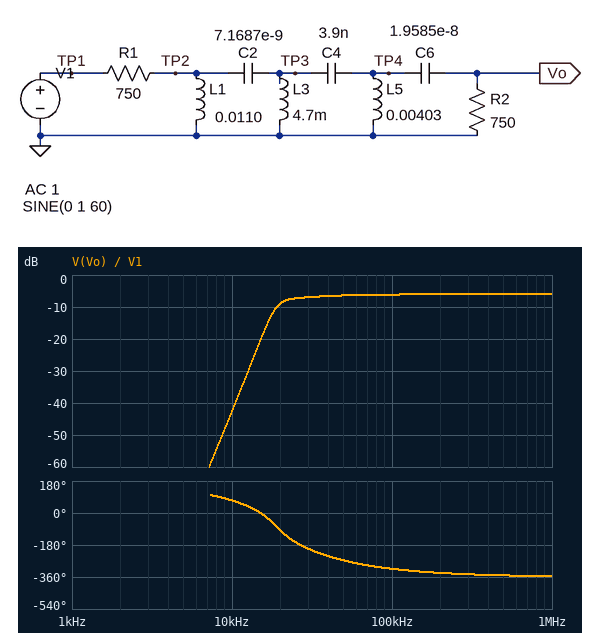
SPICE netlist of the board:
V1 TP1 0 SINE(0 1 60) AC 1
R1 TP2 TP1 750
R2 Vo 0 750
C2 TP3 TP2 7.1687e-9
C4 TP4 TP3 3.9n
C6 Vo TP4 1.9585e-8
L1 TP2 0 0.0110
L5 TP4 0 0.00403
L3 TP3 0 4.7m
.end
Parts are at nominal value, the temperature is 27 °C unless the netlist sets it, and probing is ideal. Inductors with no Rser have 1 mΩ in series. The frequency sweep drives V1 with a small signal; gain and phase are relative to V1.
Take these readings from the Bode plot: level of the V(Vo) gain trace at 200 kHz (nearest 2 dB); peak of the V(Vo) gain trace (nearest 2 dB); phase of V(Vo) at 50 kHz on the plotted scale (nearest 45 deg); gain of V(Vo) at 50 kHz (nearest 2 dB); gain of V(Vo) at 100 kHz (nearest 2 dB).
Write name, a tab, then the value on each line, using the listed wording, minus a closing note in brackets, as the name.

level of the V(Vo) gain trace at 200 kHz	-6 dB
peak of the V(Vo) gain trace	-6 dB
phase of V(Vo) at 50 kHz on the plotted scale	-270 deg
gain of V(Vo) at 50 kHz	-6 dB
gain of V(Vo) at 100 kHz	-6 dB
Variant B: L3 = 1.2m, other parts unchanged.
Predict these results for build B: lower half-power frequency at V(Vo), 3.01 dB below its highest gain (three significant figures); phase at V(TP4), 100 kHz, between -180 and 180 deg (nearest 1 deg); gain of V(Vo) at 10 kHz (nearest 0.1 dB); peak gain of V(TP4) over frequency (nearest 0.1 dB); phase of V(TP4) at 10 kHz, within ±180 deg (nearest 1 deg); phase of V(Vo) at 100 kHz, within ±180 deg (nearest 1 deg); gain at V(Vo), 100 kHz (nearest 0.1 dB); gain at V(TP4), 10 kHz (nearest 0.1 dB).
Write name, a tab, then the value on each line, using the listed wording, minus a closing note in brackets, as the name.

lower half-power frequency at V(Vo), 3.01 dB below its highest gain	41.8 kHz
phase at V(TP4), 100 kHz, between -180 and 180 deg	62 deg
gain of V(Vo) at 10 kHz	-56.2 dB
peak gain of V(TP4) over frequency	-6.0 dB
phase of V(TP4) at 10 kHz, within ±180 deg	25 deg
phase of V(Vo) at 100 kHz, within ±180 deg	68 deg
gain at V(Vo), 100 kHz	-6.3 dB
gain at V(TP4), 10 kHz	-52.8 dB
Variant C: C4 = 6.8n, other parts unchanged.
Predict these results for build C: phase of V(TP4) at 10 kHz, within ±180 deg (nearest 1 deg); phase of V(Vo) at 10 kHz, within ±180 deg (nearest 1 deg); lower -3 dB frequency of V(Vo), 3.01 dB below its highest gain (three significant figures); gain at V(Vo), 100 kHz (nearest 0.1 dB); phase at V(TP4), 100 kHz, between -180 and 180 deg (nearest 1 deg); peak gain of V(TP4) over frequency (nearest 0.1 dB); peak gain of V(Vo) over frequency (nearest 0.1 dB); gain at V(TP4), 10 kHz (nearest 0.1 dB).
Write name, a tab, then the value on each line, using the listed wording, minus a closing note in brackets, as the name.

phase of V(TP4) at 10 kHz, within ±180 deg	22 deg
phase of V(Vo) at 10 kHz, within ±180 deg	69 deg
lower -3 dB frequency of V(Vo), 3.01 dB below its highest gain	15.7 kHz
gain at V(Vo), 100 kHz	-6.0 dB
phase at V(TP4), 100 kHz, between -180 and 180 deg	33 deg
peak gain of V(TP4) over frequency	-4.8 dB
peak gain of V(Vo) over frequency	-6.0 dB
gain at V(TP4), 10 kHz	-33.1 dB
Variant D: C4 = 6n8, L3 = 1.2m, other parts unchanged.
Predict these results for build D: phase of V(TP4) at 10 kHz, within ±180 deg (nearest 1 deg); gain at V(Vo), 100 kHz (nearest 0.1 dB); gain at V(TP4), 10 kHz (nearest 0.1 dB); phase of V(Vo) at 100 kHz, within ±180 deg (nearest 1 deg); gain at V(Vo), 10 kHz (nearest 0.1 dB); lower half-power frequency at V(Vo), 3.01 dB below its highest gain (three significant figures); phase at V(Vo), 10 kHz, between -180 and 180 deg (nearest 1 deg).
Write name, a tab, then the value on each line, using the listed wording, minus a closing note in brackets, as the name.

phase of V(TP4) at 10 kHz, within ±180 deg	24 deg
gain at V(Vo), 100 kHz	-6.5 dB
gain at V(TP4), 10 kHz	-47.3 dB
phase of V(Vo) at 100 kHz, within ±180 deg	60 deg
gain at V(Vo), 10 kHz	-50.7 dB
lower half-power frequency at V(Vo), 3.01 dB below its highest gain	36.1 kHz
phase at V(Vo), 10 kHz, between -180 and 180 deg	71 deg
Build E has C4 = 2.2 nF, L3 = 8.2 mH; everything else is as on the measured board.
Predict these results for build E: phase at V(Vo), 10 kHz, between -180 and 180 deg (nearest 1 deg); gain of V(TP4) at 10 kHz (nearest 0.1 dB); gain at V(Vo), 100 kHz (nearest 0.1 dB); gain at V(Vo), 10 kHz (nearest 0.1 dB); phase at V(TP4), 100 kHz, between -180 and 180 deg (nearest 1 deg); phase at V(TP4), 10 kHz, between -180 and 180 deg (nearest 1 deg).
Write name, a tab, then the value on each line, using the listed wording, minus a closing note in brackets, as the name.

phase at V(Vo), 10 kHz, between -180 and 180 deg	69 deg
gain of V(TP4) at 10 kHz	-38.3 dB
gain at V(Vo), 100 kHz	-6.7 dB
gain at V(Vo), 10 kHz	-41.7 dB
phase at V(TP4), 100 kHz, between -180 and 180 deg	48 deg
phase at V(TP4), 10 kHz, between -180 and 180 deg	21 deg
